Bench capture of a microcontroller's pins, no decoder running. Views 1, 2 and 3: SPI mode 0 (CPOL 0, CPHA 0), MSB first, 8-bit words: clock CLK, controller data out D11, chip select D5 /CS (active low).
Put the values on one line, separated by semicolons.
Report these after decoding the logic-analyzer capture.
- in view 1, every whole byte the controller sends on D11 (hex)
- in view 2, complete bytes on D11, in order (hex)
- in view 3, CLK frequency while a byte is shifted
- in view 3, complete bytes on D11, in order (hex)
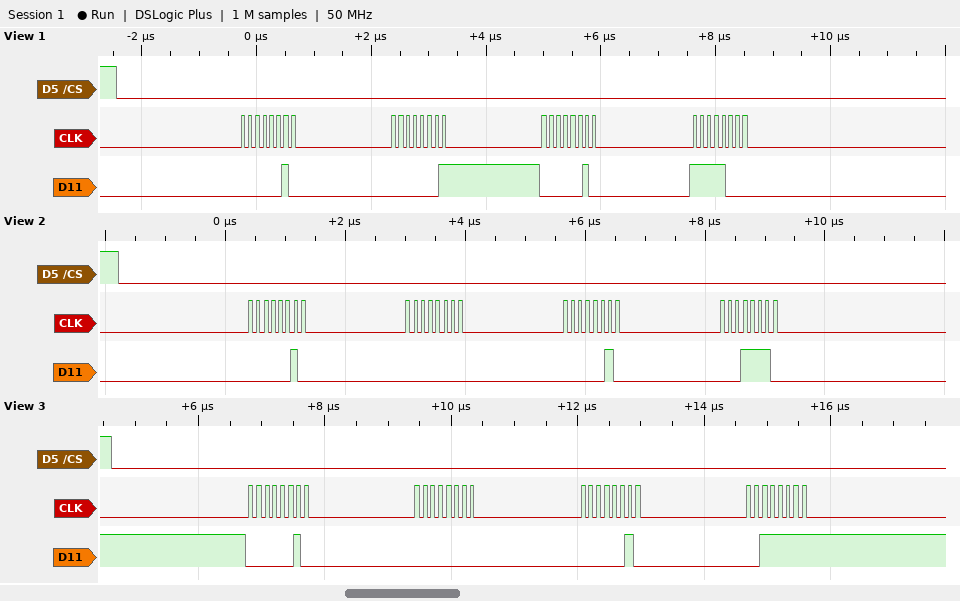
0x02 0x01 0x02 0xF8; 02 00 02 1E; 8 MHz; 02 00 02 3F
